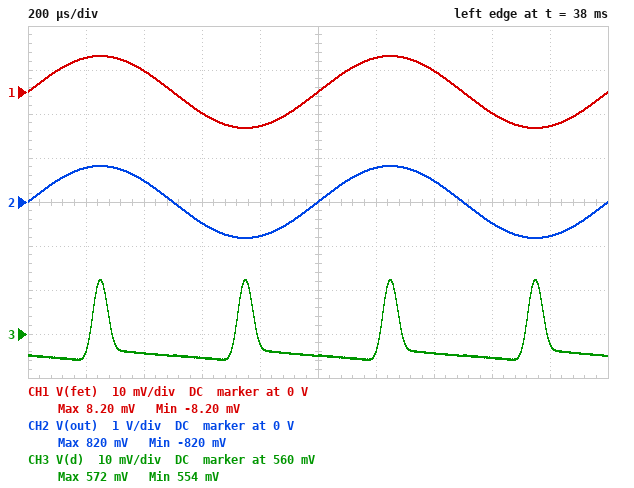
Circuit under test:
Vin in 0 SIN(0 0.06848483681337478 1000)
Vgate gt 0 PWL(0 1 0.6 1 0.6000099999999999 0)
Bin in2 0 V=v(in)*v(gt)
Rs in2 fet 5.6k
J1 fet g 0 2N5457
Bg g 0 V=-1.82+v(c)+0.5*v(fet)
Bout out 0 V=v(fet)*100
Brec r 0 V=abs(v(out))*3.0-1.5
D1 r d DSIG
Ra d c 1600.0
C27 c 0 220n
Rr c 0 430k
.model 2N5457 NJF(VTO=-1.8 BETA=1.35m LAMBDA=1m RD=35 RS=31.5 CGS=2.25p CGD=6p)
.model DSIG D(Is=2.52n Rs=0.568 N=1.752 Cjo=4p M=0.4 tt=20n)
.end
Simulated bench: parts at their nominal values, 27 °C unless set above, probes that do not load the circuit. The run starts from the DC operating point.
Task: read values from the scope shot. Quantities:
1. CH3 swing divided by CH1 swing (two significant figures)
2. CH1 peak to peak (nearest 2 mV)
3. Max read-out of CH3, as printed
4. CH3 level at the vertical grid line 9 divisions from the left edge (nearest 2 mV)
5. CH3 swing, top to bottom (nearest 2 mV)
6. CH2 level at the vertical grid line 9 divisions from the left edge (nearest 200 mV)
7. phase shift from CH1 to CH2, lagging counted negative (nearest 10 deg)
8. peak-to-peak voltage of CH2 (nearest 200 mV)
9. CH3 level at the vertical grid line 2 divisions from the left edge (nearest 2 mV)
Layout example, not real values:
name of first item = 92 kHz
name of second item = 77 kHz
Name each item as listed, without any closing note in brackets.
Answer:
CH3 swing divided by CH1 swing = 1.1
CH1 peak to peak = 16 mV
Max read-out of CH3, as printed = 572 mV
CH3 level at the vertical grid line 9 divisions from the left edge = 558 mV
CH3 swing, top to bottom = 18 mV
CH2 level at the vertical grid line 9 divisions from the left edge = -800 mV
phase shift from CH1 to CH2, lagging counted negative = 0 deg
peak-to-peak voltage of CH2 = 1.6 V
CH3 level at the vertical grid line 2 divisions from the left edge = 556 mV
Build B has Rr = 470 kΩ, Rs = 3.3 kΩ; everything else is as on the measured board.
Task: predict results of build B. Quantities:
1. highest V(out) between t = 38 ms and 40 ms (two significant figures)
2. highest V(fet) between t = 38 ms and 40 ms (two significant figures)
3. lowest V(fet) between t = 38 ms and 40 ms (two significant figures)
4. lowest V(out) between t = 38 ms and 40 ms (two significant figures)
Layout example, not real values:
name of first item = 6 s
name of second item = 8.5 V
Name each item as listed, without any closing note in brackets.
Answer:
highest V(out) between t = 38 ms and 40 ms = 920 mV
highest V(fet) between t = 38 ms and 40 ms = 9.2 mV
lowest V(fet) between t = 38 ms and 40 ms = -9.2 mV
lowest V(out) between t = 38 ms and 40 ms = -920 mV
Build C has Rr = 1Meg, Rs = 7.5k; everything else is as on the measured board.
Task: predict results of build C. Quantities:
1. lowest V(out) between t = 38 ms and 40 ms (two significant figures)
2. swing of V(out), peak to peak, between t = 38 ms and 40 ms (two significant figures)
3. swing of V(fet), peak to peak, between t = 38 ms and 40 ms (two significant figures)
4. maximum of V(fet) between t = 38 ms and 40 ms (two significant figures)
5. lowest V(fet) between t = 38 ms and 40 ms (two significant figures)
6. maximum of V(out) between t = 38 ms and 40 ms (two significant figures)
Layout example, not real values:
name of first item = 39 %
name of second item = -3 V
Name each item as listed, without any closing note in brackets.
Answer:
lowest V(out) between t = 38 ms and 40 ms = -760 mV
swing of V(out), peak to peak, between t = 38 ms and 40 ms = 1.5 V
swing of V(fet), peak to peak, between t = 38 ms and 40 ms = 15 mV
maximum of V(fet) between t = 38 ms and 40 ms = 7.6 mV
lowest V(fet) between t = 38 ms and 40 ms = -7.6 mV
maximum of V(out) between t = 38 ms and 40 ms = 760 mV
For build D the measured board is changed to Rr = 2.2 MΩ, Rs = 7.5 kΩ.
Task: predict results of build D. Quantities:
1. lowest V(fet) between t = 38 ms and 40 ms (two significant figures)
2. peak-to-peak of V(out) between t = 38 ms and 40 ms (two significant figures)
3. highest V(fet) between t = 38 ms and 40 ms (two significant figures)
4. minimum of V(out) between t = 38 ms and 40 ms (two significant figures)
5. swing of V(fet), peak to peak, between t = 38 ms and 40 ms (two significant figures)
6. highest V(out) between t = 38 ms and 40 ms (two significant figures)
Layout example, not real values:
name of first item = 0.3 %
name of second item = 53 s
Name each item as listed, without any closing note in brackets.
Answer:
lowest V(fet) between t = 38 ms and 40 ms = -7.5 mV
peak-to-peak of V(out) between t = 38 ms and 40 ms = 1.5 V
highest V(fet) between t = 38 ms and 40 ms = 7.5 mV
minimum of V(out) between t = 38 ms and 40 ms = -750 mV
swing of V(fet), peak to peak, between t = 38 ms and 40 ms = 15 mV
highest V(out) between t = 38 ms and 40 ms = 750 mV
